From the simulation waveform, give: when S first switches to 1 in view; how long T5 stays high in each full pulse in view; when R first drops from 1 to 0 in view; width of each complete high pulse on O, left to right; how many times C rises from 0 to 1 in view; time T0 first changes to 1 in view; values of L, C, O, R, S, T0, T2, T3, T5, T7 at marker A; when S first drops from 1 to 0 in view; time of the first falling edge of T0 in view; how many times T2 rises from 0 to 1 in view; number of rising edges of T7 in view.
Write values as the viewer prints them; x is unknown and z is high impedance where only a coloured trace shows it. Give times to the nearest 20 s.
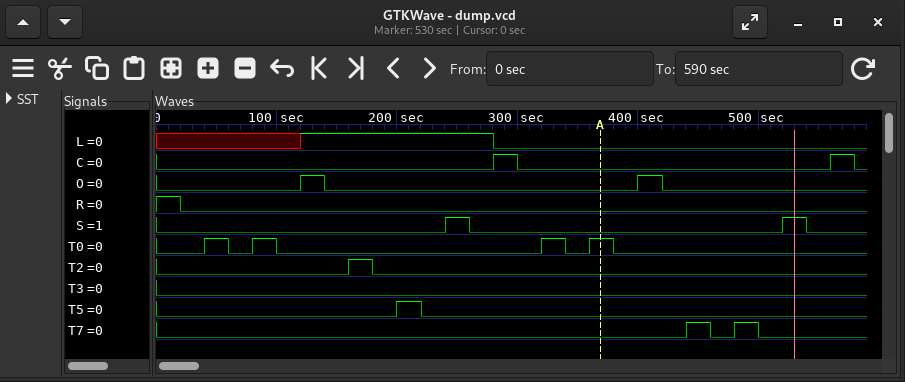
240 s
20 s
20 s
20 s, 20 s
2
40 s
L=0, C=0, O=0, R=0, S=0, T0=1, T2=0, T3=0, T5=0, T7=0
260 s
60 s
1
2
